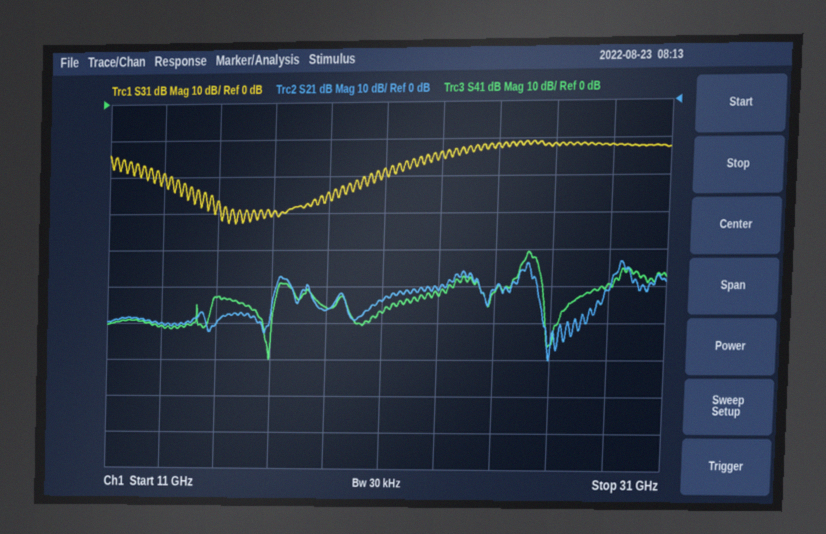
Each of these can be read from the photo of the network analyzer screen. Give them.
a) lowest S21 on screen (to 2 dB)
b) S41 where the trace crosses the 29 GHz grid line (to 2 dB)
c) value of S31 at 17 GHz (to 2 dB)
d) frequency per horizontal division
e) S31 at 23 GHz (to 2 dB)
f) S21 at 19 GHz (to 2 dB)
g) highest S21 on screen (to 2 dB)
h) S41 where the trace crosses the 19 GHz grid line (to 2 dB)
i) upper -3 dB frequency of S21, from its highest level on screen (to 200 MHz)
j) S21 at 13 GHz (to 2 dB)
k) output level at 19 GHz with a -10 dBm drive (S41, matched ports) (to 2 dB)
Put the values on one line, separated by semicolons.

-70 dB; -50 dB; -30 dB; 2 GHz; -14 dB; -56 dB; -44 dB; -56 dB; 29.8 GHz; -60 dB; -66 dBm
